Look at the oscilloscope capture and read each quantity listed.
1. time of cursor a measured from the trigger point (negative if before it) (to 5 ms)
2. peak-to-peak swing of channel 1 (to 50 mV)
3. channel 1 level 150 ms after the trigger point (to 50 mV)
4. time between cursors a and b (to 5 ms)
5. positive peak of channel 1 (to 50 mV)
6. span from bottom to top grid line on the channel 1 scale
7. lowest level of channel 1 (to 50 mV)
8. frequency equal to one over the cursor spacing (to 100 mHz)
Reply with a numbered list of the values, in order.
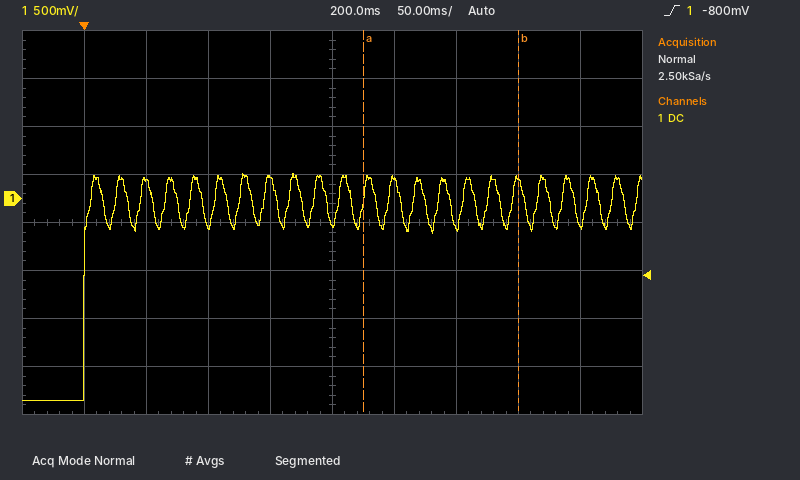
1. +225 ms
2. 2.35 V
3. 200 mV
4. 125 ms
5. 250 mV
6. 4 V
7. -2.10 V
8. 8.0 Hz
